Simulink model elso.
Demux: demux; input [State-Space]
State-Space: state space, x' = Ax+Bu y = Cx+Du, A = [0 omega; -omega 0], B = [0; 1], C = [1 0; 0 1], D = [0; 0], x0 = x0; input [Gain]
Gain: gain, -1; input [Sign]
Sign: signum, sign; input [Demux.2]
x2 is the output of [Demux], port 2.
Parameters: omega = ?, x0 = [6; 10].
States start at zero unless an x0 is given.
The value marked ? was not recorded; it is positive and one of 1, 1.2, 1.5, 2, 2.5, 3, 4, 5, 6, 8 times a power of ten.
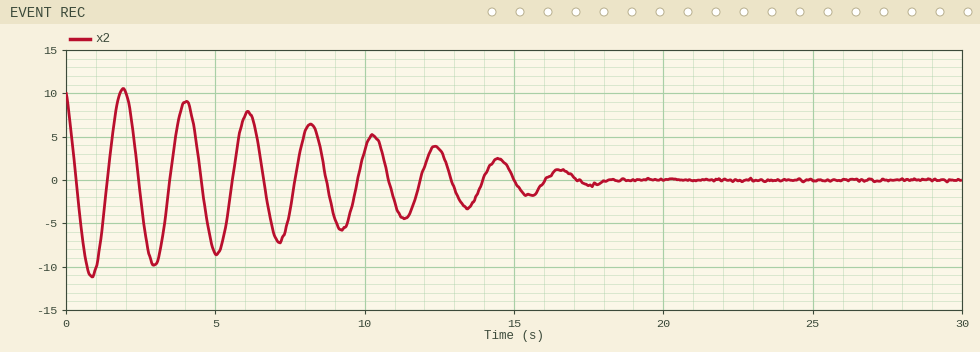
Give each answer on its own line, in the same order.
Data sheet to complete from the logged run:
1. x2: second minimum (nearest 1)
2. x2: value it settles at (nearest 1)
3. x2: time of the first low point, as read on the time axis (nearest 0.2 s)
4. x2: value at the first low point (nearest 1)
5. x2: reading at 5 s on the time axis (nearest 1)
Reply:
-10
0
0.8 s
-11
-8
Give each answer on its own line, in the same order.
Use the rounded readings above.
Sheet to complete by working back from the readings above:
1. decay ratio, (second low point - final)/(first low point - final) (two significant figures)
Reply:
0.91
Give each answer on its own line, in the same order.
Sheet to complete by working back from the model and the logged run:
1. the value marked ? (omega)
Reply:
3
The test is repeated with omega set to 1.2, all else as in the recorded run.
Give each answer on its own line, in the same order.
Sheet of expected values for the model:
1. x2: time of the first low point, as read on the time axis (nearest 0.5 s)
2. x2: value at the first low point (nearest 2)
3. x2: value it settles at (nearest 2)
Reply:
2.0 s
-10
0
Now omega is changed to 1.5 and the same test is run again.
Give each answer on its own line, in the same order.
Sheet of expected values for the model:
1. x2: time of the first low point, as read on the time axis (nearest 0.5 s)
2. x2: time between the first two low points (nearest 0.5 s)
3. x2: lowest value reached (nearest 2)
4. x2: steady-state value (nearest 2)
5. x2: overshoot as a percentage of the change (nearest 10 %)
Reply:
1.5 s
4.0 s
-10
0
110 %
